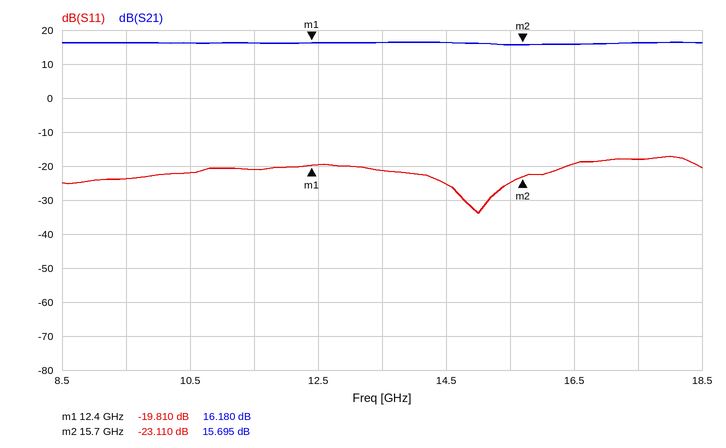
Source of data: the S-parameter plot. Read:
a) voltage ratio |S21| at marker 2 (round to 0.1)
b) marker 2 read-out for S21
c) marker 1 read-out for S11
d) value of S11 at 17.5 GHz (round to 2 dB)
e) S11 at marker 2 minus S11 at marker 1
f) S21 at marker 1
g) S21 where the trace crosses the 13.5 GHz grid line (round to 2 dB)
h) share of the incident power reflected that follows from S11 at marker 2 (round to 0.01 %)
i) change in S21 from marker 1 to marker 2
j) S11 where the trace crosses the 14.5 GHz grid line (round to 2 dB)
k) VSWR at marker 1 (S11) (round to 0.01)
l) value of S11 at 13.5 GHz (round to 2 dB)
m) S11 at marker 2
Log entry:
6.1
15.695 dB
-19.810 dB
-18 dB
-3.300 dB
16.180 dB
16 dB
0.49 %
-0.485 dB
-26 dB
1.23
-22 dB
-23.110 dB
